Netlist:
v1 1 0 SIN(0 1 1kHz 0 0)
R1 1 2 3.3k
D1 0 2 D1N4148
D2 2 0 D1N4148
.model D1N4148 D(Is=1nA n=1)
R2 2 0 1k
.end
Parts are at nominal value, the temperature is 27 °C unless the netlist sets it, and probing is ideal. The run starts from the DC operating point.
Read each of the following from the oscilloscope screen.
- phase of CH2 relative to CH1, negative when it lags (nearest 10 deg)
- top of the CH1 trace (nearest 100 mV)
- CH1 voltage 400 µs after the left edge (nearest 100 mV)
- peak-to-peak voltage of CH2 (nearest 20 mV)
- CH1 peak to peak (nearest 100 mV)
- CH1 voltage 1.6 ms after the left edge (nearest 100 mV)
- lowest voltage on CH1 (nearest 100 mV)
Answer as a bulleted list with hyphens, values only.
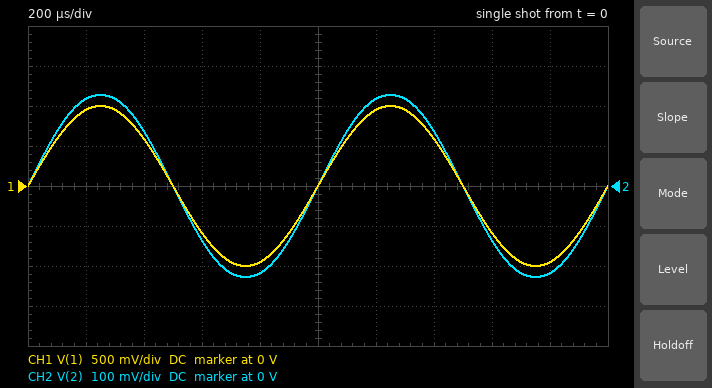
- 0 deg
- 1.0 V
- 600 mV
- 460 mV
- 2.0 V
- -600 mV
- -1.0 V
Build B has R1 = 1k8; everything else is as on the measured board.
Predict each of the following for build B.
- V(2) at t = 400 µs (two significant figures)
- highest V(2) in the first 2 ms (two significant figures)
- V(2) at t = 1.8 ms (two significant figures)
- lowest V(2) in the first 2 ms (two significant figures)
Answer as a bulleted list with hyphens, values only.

- 210 mV
- 300 mV
- -290 mV
- -300 mV
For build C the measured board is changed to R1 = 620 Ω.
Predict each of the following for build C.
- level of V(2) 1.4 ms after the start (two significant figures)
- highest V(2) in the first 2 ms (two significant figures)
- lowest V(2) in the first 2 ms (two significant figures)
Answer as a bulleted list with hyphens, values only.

- 310 mV
- 350 mV
- -350 mV
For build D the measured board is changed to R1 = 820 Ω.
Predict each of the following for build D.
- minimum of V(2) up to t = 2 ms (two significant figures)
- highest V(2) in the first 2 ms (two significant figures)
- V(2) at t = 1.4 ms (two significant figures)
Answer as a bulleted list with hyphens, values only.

- -340 mV
- 340 mV
- 290 mV
